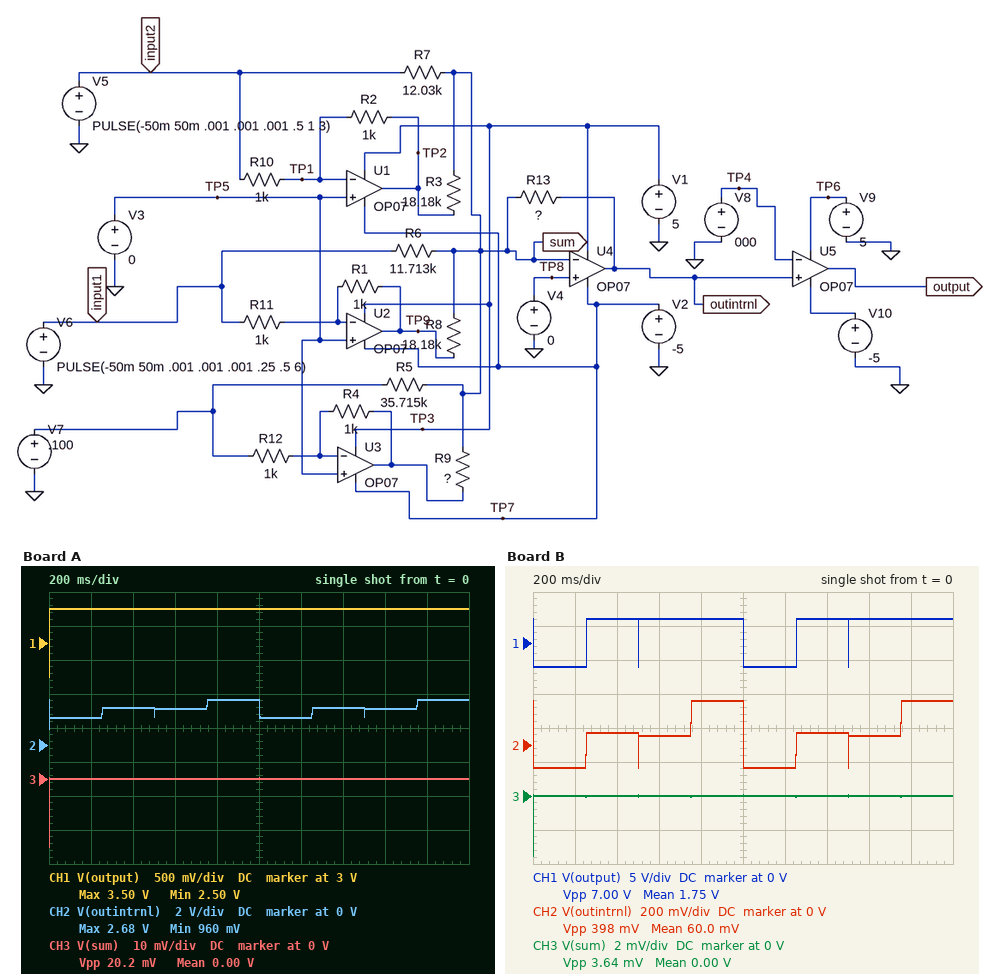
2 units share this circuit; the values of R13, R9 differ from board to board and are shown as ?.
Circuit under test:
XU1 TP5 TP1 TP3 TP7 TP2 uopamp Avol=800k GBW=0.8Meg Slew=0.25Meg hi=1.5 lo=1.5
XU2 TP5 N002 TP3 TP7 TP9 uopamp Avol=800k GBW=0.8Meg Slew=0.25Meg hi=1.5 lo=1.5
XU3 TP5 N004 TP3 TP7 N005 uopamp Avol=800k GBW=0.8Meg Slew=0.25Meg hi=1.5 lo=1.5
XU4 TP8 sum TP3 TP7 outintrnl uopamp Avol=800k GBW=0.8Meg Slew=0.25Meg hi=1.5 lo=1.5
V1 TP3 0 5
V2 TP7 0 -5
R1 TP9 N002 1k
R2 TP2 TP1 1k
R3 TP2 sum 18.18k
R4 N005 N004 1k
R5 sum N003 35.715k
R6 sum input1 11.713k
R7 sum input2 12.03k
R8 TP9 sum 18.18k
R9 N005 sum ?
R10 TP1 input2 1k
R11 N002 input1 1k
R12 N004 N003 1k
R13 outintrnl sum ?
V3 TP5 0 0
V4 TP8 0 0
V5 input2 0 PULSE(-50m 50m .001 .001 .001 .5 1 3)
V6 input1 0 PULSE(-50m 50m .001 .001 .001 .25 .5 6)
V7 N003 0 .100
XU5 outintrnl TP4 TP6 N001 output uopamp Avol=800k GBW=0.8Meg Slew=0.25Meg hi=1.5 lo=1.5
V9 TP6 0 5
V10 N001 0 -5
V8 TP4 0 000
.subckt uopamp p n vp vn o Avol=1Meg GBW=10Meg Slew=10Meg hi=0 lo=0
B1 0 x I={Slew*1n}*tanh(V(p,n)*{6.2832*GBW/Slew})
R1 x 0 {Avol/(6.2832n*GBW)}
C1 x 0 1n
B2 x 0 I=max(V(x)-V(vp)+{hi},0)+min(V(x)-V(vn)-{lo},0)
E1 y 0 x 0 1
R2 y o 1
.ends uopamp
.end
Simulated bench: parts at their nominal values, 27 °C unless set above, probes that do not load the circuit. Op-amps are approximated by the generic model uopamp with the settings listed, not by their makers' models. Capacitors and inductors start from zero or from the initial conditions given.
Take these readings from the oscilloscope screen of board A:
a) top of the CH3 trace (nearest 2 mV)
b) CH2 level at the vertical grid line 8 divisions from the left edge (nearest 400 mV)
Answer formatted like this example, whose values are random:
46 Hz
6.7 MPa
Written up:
0 V
2.0 V
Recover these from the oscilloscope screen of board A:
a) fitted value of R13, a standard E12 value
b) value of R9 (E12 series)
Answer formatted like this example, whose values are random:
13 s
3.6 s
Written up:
180 kΩ
6.8 kΩ
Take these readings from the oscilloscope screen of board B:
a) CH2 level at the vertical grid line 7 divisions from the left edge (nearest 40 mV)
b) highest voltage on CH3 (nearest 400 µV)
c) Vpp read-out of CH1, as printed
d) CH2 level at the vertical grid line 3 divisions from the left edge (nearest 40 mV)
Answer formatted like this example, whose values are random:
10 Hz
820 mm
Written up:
80 mV
0 V
7.00 V
40 mV
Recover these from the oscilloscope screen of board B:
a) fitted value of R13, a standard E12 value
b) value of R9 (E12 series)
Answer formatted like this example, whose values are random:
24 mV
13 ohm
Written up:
68 kΩ
27 kΩ
